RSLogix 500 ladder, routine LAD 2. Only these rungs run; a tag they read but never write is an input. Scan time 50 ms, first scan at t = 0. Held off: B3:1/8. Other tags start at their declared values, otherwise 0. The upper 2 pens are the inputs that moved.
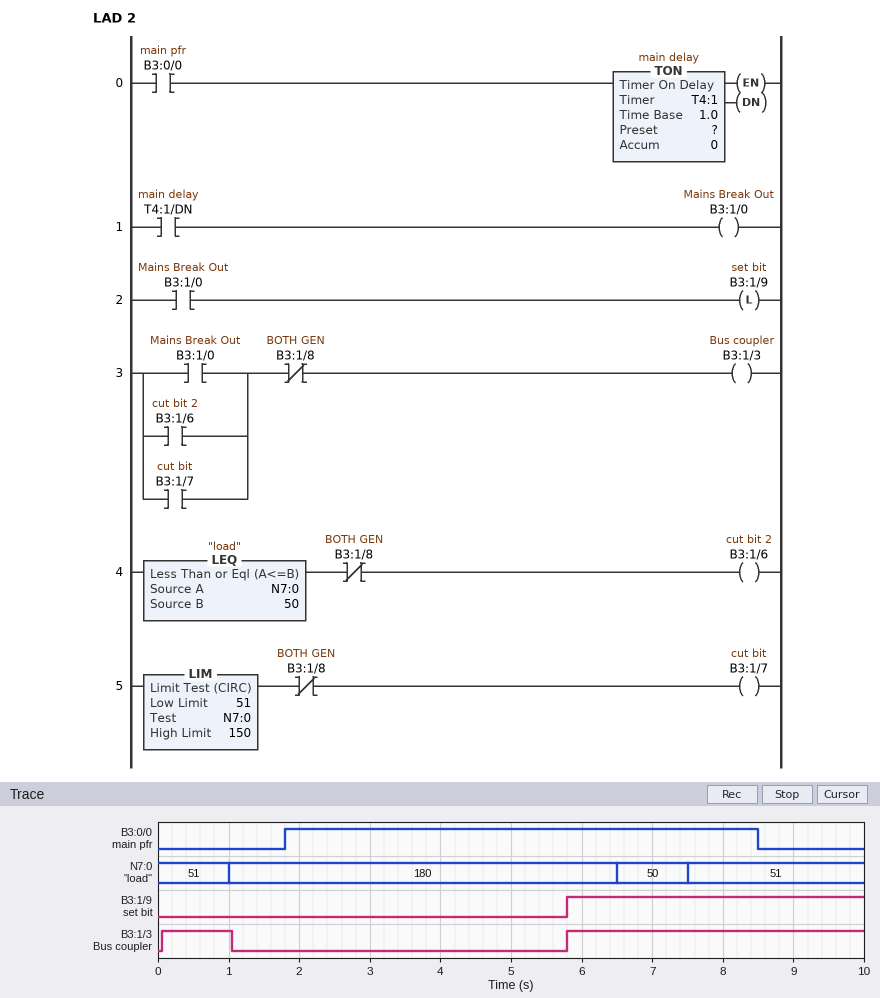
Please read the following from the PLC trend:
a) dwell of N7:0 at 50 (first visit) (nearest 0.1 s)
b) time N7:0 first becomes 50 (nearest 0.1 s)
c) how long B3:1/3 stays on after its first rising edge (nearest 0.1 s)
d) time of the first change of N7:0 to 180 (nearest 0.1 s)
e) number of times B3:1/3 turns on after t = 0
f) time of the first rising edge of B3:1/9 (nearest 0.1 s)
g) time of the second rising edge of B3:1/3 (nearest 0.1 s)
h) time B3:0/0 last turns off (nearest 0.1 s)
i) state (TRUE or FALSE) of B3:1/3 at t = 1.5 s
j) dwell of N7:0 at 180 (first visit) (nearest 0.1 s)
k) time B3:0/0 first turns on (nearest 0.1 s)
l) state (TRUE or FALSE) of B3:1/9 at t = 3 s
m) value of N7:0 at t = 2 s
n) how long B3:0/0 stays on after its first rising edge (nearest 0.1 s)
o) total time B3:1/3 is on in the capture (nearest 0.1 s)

1.0 s
6.5 s
1.0 s
1.0 s
2
5.8 s
5.8 s
8.5 s
FALSE
5.5 s
1.8 s
FALSE
180
6.7 s
5.2 s
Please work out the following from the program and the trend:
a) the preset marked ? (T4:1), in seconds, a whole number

4 s
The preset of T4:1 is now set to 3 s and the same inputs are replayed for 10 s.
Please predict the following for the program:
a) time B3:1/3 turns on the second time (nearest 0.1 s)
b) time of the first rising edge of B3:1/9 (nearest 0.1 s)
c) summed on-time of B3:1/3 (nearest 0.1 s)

4.8 s
4.8 s
6.2 s
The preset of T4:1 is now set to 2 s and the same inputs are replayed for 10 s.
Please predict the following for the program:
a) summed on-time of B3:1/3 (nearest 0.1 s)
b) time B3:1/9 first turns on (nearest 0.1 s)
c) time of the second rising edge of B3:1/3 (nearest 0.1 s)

7.2 s
3.8 s
3.8 s
